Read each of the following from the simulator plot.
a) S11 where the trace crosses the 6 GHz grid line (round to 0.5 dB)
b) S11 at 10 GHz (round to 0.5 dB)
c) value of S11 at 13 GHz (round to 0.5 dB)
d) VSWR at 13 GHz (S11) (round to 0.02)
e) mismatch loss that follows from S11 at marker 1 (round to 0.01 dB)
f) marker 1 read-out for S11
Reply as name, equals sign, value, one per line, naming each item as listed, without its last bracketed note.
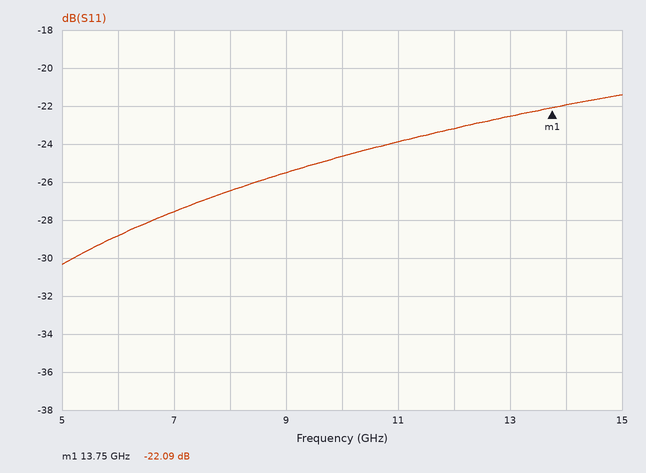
S11 where the trace crosses the 6 GHz grid line = -29.0 dB
S11 at 10 GHz = -24.5 dB
value of S11 at 13 GHz = -22.5 dB
VSWR at 13 GHz (S11) = 1.16
mismatch loss that follows from S11 at marker 1 = 0.03 dB
marker 1 read-out for S11 = -22.09 dB
